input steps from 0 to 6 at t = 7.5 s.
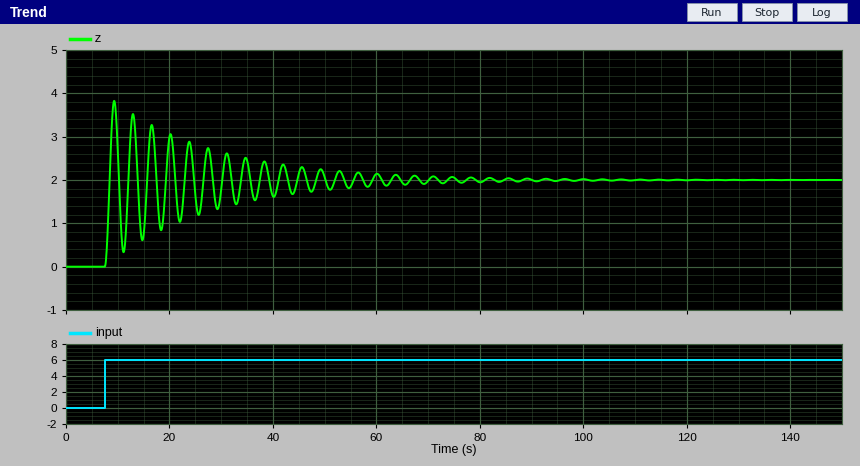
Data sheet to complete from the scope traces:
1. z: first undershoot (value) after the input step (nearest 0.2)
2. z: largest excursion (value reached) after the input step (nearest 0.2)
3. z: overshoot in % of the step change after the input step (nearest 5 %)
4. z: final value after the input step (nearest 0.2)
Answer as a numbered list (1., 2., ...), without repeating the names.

1. 0.4
2. 3.8
3. 90 %
4. 2.0
